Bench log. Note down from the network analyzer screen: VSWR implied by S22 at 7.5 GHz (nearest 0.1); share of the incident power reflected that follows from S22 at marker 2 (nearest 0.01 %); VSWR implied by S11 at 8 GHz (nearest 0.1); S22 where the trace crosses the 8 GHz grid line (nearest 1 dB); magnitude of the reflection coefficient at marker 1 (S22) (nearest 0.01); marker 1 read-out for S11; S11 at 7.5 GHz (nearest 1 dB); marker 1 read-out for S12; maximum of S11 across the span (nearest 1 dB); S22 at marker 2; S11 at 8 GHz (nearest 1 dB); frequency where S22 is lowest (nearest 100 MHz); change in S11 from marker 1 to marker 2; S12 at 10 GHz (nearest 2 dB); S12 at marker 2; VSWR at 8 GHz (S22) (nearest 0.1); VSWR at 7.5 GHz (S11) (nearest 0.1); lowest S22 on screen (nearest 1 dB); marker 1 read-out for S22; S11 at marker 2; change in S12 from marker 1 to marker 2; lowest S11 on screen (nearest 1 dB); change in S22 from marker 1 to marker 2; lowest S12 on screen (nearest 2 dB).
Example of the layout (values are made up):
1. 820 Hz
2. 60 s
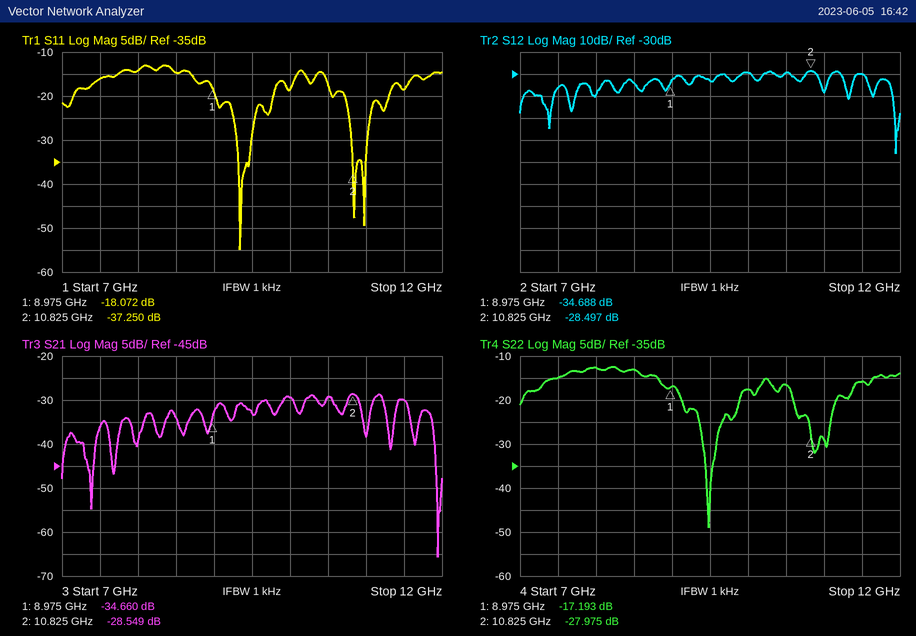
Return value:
1. 1.4
2. 0.16 %
3. 1.5
4. -13 dB
5. 0.14
6. -18.072 dB
7. -16 dB
8. -34.688 dB
9. -13 dB
10. -27.975 dB
11. -14 dB
12. 9.5 GHz
13. -19.178 dB
14. -30 dB
15. -28.497 dB
16. 1.6
17. 1.4
18. -49 dB
19. -17.193 dB
20. -37.250 dB
21. 6.191 dB
22. -55 dB
23. -10.782 dB
24. -66 dB
